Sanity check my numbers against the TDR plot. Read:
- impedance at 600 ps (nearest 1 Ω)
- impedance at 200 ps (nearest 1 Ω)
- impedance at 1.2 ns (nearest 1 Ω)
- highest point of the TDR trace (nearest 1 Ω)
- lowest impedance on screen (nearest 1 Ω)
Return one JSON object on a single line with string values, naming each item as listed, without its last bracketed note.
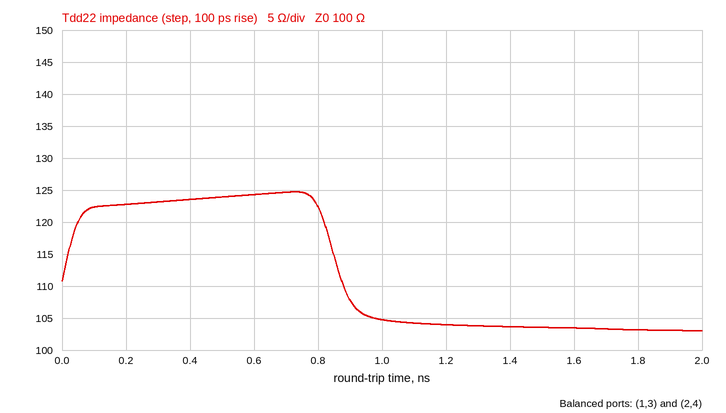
{"impedance at 600 ps": "124 Ω", "impedance at 200 ps": "123 Ω", "impedance at 1.2 ns": "104 Ω", "highest point of the TDR trace": "125 Ω", "lowest impedance on screen": "103 Ω"}
